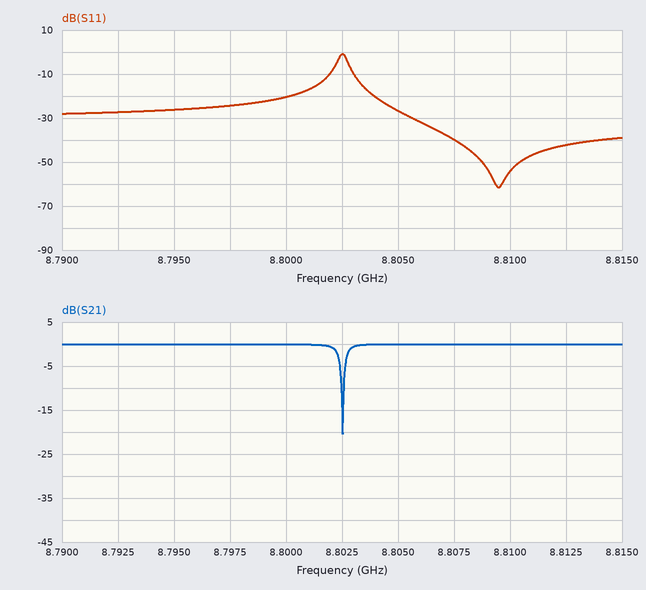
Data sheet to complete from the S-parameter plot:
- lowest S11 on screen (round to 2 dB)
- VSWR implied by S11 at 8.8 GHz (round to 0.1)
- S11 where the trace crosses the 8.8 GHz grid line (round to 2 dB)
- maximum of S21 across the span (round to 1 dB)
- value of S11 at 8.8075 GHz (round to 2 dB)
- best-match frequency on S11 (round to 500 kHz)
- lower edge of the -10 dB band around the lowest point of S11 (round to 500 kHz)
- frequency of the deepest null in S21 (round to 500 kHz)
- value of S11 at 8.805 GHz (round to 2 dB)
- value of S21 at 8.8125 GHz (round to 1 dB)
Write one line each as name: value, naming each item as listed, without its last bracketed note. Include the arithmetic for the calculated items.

lowest S11 on screen: -62 dB
VSWR implied by S11 at 8.8 GHz: |Γ| = 10^(-20/20) = 0.1000; VSWR = (1 + 0.1000)/(1 − 0.1000) ≈ 1.2
S11 where the trace crosses the 8.8 GHz grid line: -20 dB
maximum of S21 across the span: 0 dB
value of S11 at 8.8075 GHz: -40 dB
best-match frequency on S11: 8.8095 GHz
lower edge of the -10 dB band around the lowest point of S11: 8.8030 GHz
frequency of the deepest null in S21: 8.8025 GHz
value of S11 at 8.805 GHz: -26 dB
value of S21 at 8.8125 GHz: 0 dB
